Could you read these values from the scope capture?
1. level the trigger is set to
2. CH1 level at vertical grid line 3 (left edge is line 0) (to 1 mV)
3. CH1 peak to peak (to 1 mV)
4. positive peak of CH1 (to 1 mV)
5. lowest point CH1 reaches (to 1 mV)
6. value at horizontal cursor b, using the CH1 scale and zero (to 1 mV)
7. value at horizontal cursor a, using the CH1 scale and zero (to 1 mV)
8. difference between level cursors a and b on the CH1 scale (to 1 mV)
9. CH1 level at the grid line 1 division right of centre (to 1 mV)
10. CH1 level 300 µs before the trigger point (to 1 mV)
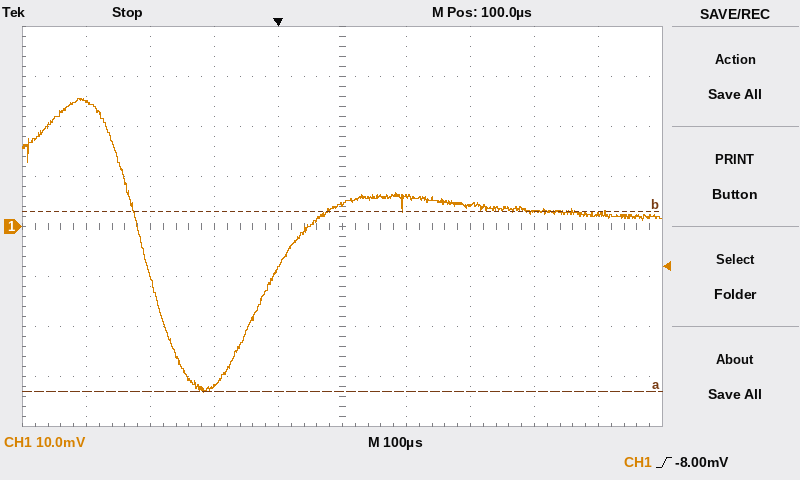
-8.00 mV
-32 mV
59 mV
26 mV
-33 mV
3 mV
-33 mV
36 mV
6 mV
25 mV
